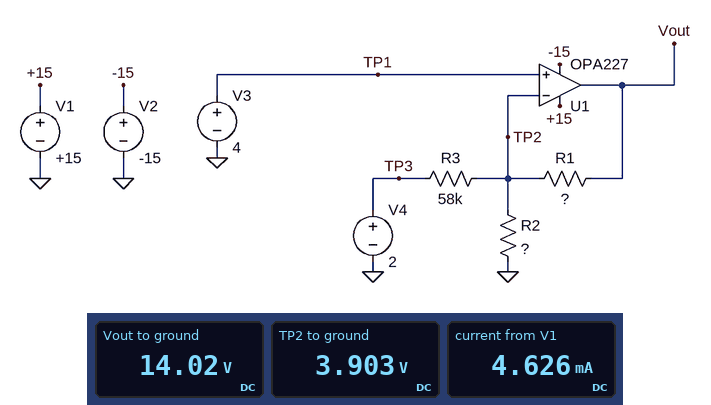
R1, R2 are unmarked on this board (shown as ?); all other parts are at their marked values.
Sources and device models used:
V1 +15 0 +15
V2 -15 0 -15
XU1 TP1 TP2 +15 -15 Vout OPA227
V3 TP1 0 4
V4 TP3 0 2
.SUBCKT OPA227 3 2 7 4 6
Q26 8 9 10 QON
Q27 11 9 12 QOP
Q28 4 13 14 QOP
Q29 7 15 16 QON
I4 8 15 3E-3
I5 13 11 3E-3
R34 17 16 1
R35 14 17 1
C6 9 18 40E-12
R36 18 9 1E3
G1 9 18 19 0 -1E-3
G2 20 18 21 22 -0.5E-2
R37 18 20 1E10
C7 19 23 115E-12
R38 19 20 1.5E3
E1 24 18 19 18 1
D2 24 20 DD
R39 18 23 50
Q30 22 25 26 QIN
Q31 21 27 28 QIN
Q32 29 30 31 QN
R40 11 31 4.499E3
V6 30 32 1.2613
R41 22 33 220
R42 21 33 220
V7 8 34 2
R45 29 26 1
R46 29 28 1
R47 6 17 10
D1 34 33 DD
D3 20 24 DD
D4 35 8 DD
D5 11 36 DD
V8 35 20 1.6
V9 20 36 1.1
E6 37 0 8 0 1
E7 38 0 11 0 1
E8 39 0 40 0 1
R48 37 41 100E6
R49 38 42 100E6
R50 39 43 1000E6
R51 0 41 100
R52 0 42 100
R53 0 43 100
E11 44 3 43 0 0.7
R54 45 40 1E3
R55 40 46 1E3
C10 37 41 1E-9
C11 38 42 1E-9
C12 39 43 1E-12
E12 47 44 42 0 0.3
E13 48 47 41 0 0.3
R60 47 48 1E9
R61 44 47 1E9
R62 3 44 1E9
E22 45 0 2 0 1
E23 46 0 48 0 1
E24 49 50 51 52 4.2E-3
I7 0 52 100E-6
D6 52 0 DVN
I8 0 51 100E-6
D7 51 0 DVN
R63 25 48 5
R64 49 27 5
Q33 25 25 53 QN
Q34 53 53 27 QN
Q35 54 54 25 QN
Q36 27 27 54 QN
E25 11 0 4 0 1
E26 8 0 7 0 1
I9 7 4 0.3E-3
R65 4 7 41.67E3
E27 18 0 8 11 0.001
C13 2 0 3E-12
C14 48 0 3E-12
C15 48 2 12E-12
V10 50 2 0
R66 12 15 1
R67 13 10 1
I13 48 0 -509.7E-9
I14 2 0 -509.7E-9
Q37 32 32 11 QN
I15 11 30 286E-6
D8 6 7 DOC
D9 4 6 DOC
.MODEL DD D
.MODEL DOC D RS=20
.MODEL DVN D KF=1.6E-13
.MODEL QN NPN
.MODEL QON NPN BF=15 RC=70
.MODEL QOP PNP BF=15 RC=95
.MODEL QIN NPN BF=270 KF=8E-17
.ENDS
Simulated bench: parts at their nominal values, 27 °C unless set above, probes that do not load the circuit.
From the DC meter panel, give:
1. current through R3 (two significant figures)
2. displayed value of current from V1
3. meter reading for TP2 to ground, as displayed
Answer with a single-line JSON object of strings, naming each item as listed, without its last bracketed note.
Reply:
{"current through R3": "33 µA", "displayed value of current from V1": "4.626 mA", "meter reading for TP2 to ground, as displayed": "3.903 V"}
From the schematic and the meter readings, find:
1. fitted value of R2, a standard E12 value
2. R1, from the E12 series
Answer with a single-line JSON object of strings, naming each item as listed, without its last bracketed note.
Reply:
{"fitted value of R2, a standard E12 value": "2.2 kΩ", "R1, from the E12 series": "5.6 kΩ"}
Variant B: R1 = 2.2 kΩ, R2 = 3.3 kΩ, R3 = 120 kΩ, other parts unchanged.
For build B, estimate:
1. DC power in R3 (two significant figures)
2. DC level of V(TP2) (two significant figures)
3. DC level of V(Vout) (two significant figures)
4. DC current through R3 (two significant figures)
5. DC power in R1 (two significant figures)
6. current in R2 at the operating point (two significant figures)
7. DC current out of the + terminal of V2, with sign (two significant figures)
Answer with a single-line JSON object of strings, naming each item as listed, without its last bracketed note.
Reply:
{"DC power in R3": "33 µW", "DC level of V(TP2)": "4.0 V", "DC level of V(Vout)": "6.7 V", "DC current through R3": "17 µA", "DC power in R1": "3.3 mW", "current in R2 at the operating point": "1.2 mA", "DC current out of the + terminal of V2, with sign": "-3.1 mA"}
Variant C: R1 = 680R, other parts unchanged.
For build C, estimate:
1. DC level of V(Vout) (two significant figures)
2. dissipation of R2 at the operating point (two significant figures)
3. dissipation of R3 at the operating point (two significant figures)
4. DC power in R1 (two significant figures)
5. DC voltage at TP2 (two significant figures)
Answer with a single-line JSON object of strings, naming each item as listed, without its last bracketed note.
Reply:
{"DC level of V(Vout)": "5.3 V", "dissipation of R2 at the operating point": "7.3 mW", "dissipation of R3 at the operating point": "69 µW", "DC power in R1": "2.3 mW", "DC voltage at TP2": "4.0 V"}
